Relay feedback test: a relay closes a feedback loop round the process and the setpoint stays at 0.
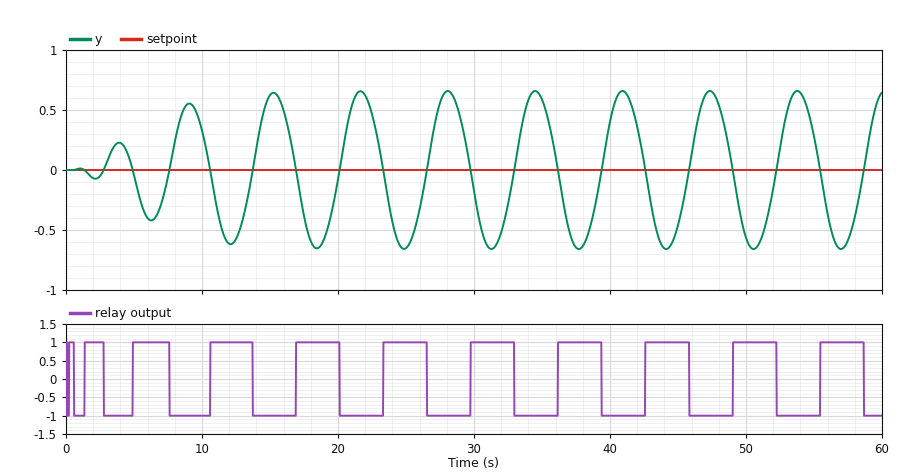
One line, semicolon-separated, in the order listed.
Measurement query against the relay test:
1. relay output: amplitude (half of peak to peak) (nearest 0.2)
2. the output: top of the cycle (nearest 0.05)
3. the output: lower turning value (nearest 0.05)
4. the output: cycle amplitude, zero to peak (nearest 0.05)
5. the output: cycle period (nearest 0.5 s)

1.0; 0.65; -0.65; 0.65; 6.5 s
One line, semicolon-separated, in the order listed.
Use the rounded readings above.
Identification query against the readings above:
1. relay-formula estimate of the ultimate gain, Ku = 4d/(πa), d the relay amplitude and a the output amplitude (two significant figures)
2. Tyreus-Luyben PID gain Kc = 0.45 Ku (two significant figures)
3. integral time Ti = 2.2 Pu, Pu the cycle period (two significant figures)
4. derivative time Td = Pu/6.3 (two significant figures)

2.0; 0.90; 14 s; 1.0 s
